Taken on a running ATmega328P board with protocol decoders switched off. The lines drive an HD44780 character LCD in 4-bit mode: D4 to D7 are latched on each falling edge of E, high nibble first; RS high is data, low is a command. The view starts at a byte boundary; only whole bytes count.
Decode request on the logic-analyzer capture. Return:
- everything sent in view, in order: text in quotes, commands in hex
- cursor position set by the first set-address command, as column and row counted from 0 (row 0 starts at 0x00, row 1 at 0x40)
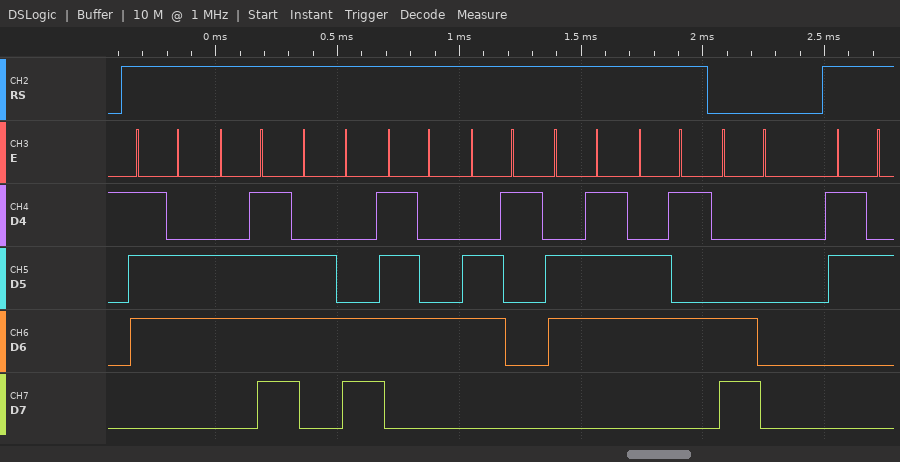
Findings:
"voltage" 0xC0 "2"
column 0, row 1
